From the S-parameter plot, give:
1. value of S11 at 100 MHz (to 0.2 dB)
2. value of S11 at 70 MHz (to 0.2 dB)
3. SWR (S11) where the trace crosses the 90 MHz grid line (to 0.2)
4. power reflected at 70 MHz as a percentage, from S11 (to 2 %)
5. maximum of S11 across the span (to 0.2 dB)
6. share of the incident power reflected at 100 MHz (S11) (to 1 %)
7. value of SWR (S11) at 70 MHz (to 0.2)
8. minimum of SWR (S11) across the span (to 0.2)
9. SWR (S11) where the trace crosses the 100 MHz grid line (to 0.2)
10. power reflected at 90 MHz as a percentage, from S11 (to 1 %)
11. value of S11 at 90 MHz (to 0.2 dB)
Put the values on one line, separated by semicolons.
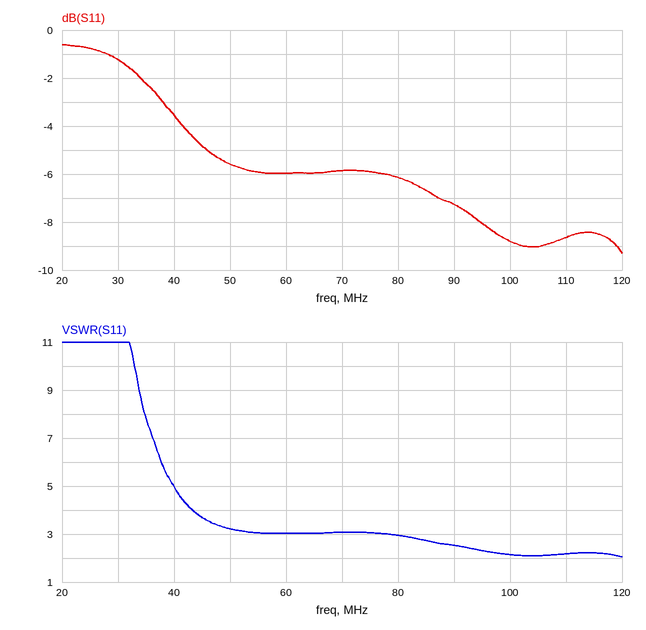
-8.8 dB; -5.8 dB; 2.6; 26 %; -0.6 dB; 13 %; 3.0; 2.0; 2.2; 19 %; -7.2 dB
